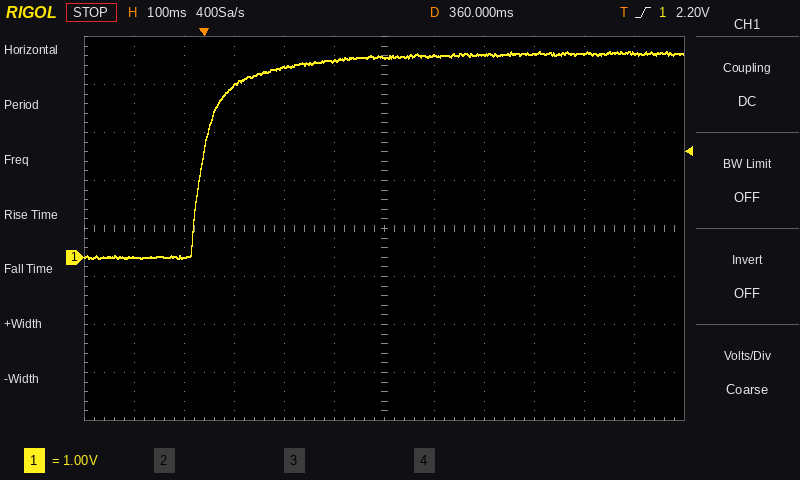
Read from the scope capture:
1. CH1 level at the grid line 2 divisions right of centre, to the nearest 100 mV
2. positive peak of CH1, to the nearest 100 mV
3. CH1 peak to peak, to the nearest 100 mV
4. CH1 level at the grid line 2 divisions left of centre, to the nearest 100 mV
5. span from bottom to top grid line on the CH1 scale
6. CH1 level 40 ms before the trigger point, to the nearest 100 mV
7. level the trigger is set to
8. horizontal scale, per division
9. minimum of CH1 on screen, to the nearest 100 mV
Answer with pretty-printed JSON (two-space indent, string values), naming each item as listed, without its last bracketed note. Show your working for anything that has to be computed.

{
  "CH1 level at the grid line 2 divisions right of centre, to the nearest 100 mV": "4.2 V",
  "positive peak of CH1, to the nearest 100 mV": "4.3 V",
  "CH1 peak to peak, to the nearest 100 mV": "4.3 V − (0.0 V) = 4.3 V",
  "CH1 level at the grid line 2 divisions left of centre, to the nearest 100 mV": "4.0 V",
  "span from bottom to top grid line on the CH1 scale": "8 V",
  "CH1 level 40 ms before the trigger point, to the nearest 100 mV": "0.0 V",
  "level the trigger is set to": "2.20 V",
  "horizontal scale, per division": "100 ms",
  "minimum of CH1 on screen, to the nearest 100 mV": "0.0 V"
}
